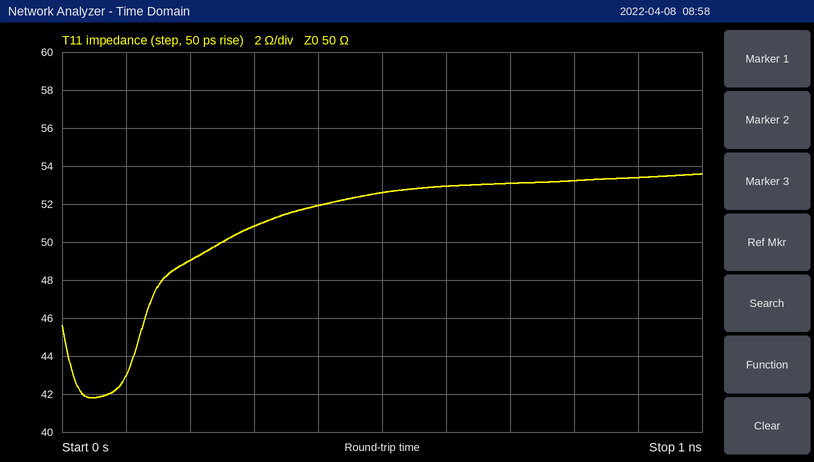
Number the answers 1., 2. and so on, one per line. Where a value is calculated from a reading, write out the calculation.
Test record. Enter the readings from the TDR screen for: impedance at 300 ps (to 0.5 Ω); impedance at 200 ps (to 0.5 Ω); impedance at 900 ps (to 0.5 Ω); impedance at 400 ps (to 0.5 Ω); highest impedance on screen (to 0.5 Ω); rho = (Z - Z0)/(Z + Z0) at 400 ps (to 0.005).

1. 51.0 Ω
2. 49.0 Ω
3. 53.5 Ω
4. 52.0 Ω
5. 53.5 Ω
6. (52 − 50)/(52 + 50) ≈ +0.020
